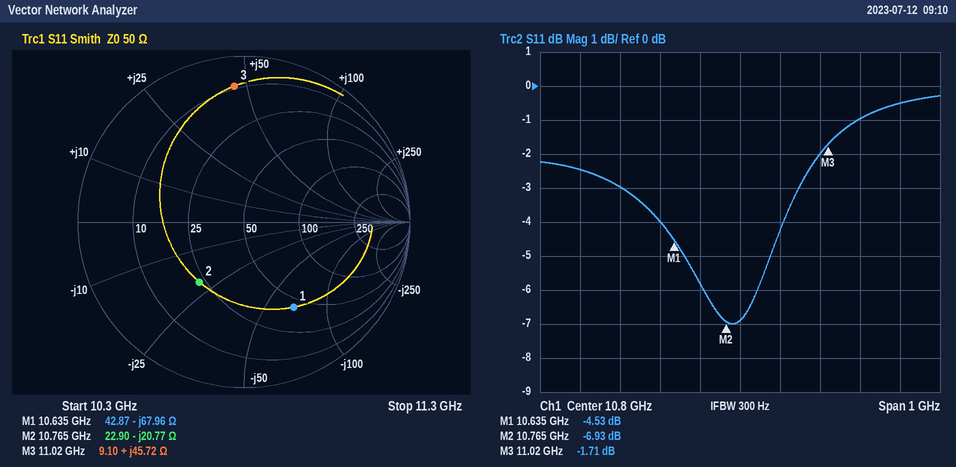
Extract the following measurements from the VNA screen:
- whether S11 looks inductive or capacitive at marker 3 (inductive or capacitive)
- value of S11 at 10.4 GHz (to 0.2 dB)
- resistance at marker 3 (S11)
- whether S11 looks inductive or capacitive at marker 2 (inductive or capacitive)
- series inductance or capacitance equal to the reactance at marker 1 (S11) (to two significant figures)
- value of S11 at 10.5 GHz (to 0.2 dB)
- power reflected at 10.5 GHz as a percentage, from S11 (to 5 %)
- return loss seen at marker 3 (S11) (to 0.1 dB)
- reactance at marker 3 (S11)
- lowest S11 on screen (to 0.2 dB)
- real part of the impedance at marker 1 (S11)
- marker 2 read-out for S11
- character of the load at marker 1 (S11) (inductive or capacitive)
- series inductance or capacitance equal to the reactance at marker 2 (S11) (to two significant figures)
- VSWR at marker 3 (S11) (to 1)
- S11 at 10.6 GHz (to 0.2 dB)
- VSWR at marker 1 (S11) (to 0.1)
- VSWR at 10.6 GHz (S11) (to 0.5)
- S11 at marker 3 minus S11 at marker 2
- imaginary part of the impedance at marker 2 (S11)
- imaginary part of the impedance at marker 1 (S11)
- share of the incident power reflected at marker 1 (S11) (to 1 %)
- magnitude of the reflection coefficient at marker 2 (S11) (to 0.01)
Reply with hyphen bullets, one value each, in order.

- inductive
- -2.4 dB
- 9.10 Ω
- capacitive
- 220 fF
- -3.0 dB
- 50 %
- 1.7 dB
- +45.72 Ω
- -7.0 dB
- 42.87 Ω
- -6.93 dB
- capacitive
- 710 fF
- 10
- -4.0 dB
- 3.9
- 4.5
- 5.22 dB
- -20.77 Ω
- -67.96 Ω
- 35 %
- 0.45
